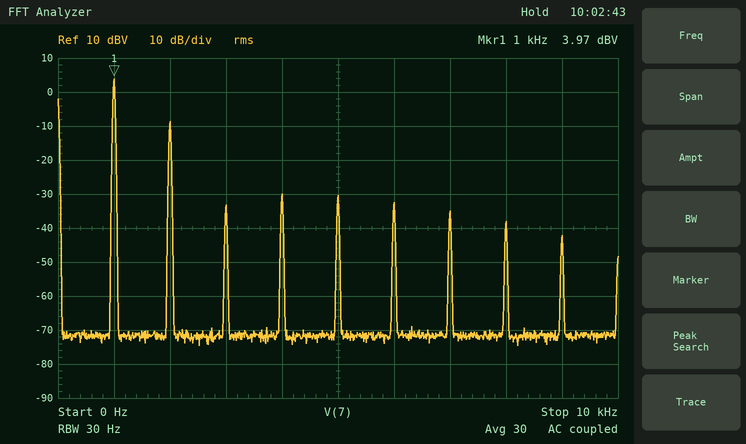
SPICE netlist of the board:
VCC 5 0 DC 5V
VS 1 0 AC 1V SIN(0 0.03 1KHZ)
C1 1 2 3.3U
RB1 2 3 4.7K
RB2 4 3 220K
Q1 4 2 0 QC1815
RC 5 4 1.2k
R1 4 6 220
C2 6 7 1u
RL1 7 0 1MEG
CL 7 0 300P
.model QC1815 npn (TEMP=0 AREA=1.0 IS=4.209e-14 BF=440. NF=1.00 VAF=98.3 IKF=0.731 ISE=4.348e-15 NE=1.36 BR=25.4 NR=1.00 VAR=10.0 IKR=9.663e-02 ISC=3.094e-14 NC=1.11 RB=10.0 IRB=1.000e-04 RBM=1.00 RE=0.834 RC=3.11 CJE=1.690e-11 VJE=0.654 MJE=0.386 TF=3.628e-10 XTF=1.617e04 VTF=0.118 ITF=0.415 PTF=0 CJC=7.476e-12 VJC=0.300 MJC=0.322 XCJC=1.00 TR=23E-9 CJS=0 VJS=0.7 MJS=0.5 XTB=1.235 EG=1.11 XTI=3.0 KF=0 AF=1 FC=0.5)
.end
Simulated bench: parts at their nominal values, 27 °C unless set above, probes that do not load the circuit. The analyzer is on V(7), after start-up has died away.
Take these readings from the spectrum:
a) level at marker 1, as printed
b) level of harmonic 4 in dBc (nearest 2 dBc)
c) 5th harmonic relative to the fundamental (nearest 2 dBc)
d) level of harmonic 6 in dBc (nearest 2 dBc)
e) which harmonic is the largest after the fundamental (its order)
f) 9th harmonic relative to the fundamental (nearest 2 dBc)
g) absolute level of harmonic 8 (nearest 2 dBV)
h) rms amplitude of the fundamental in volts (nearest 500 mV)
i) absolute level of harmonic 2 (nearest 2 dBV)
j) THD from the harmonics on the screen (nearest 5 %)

3.97 dBV
-34 dBc
-34 dBc
-36 dBc
2
-46 dBc
-38 dBV
1.5 V
-8 dBV
25 %
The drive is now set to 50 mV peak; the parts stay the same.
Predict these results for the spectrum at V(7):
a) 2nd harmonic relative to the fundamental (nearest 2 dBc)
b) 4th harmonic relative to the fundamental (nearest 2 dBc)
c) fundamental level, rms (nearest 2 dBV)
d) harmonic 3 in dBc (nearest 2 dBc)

-8 dBc
-32 dBc
4 dBV
-24 dBc
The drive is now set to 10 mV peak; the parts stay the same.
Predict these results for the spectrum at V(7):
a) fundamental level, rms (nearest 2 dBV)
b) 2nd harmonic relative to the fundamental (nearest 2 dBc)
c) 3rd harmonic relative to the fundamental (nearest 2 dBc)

-2 dBV
-22 dBc
-48 dBc
